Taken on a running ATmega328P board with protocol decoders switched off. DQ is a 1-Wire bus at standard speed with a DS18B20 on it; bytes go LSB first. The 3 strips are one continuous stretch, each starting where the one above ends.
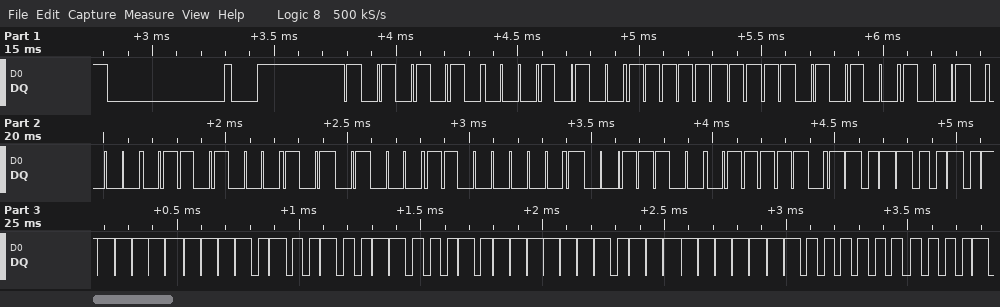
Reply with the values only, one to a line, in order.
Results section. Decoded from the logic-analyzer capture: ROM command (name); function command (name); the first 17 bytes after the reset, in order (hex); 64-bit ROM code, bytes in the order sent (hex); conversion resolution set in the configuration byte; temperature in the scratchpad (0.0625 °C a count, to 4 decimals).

Match ROM
Read Scratchpad
55 28 FF 2B 09 16 15 03 39 BE 4D FF 4B 46 7F FF 03
28 FF 2B 09 16 15 03 39
12 bits
-11.1875 °C
